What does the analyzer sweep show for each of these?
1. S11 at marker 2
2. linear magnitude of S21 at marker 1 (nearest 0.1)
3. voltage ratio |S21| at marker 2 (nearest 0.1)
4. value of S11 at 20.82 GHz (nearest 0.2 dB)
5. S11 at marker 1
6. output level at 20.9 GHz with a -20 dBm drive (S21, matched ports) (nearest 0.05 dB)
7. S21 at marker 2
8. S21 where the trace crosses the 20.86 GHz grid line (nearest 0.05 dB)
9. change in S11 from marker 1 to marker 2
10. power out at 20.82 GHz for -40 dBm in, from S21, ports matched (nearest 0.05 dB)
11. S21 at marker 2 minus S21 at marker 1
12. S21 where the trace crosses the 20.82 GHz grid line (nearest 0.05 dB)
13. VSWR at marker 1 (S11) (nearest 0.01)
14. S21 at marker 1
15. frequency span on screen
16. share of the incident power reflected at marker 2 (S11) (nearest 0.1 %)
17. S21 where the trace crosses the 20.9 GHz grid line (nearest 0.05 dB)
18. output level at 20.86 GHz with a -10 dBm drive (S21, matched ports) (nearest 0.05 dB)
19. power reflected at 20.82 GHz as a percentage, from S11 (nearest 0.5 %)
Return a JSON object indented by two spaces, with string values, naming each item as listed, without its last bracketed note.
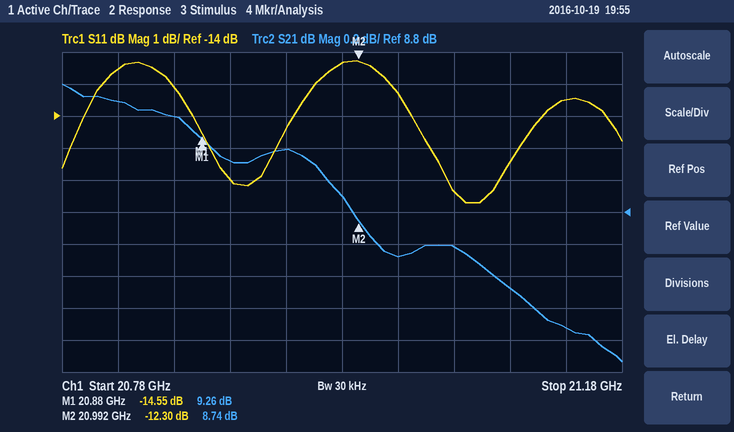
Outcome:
{
  "S11 at marker 2": "-12.30 dB",
  "linear magnitude of S21 at marker 1": "2.9",
  "voltage ratio |S21| at marker 2": "2.7",
  "value of S11 at 20.82 GHz": "-12.6 dB",
  "S11 at marker 1": "-14.55 dB",
  "output level at 20.9 GHz with a -20 dBm drive (S21, matched ports)": "-10.90 dBm",
  "S21 at marker 2": "8.74 dB",
  "S21 where the trace crosses the 20.86 GHz grid line": "9.40 dB",
  "change in S11 from marker 1 to marker 2": "2.25 dB",
  "power out at 20.82 GHz for -40 dBm in, from S21, ports matched": "-30.50 dBm",
  "S21 at marker 2 minus S21 at marker 1": "-0.52 dB",
  "S21 where the trace crosses the 20.82 GHz grid line": "9.50 dB",
  "VSWR at marker 1 (S11)": "1.46",
  "S21 at marker 1": "9.26 dB",
  "frequency span on screen": "400 MHz",
  "share of the incident power reflected at marker 2 (S11)": "5.9 %",
  "S21 where the trace crosses the 20.9 GHz grid line": "9.10 dB",
  "output level at 20.86 GHz with a -10 dBm drive (S21, matched ports)": "-0.60 dBm",
  "power reflected at 20.82 GHz as a percentage, from S11": "5.5 %"
}
